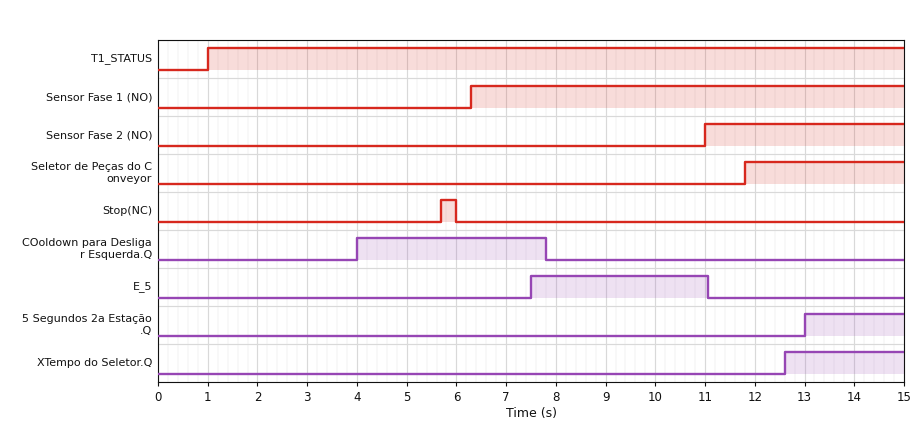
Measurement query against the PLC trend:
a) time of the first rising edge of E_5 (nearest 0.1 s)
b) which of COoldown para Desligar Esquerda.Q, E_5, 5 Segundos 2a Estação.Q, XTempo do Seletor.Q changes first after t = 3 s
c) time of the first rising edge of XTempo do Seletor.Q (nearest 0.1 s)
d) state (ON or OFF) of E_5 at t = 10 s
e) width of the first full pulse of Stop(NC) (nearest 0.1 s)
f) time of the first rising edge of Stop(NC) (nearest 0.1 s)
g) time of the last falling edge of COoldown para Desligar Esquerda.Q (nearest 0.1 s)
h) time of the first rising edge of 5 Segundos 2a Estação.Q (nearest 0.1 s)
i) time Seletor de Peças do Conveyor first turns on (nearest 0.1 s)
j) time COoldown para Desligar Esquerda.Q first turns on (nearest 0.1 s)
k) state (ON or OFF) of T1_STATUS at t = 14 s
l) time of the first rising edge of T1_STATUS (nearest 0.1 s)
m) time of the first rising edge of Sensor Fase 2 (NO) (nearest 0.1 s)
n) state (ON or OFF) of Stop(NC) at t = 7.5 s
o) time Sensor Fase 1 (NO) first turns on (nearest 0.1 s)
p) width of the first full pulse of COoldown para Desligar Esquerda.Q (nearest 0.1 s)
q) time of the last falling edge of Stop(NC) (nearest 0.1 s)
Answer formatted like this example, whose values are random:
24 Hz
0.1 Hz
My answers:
7.5 s
COoldown para Desligar Esquerda.Q
12.6 s
ON
0.3 s
5.7 s
7.8 s
13.0 s
11.8 s
4.0 s
ON
1.0 s
11.0 s
OFF
6.3 s
3.8 s
6.0 s
